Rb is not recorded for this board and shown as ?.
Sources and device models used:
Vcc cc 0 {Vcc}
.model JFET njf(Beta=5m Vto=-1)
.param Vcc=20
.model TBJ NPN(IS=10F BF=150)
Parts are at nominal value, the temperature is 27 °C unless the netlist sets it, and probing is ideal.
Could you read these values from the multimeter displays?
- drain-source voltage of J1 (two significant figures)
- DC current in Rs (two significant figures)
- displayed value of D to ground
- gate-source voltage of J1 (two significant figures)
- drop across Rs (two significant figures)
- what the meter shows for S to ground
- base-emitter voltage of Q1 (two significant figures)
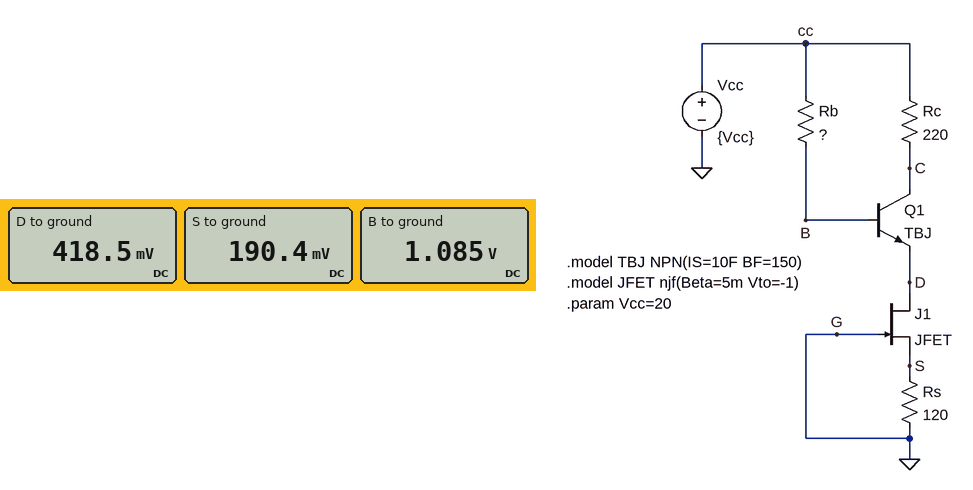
230 mV
1.6 mA
418.5 mV
-190 mV
190 mV
190.4 mV
670 mV
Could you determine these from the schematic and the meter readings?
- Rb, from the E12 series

1.8 MΩ
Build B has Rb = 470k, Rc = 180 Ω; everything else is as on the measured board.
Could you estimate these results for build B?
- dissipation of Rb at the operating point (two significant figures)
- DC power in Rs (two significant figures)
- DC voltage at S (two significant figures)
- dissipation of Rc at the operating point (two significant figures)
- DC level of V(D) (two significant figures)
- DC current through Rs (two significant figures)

130 µW
730 µW
300 mV
1.1 mW
12 V
2.5 mA
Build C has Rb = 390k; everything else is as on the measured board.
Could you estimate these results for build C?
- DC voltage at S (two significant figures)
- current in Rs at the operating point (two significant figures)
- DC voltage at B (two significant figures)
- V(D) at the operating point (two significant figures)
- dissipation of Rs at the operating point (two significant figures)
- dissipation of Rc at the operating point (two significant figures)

300 mV
2.5 mA
14 V
13 V
730 µW
1.3 mW
